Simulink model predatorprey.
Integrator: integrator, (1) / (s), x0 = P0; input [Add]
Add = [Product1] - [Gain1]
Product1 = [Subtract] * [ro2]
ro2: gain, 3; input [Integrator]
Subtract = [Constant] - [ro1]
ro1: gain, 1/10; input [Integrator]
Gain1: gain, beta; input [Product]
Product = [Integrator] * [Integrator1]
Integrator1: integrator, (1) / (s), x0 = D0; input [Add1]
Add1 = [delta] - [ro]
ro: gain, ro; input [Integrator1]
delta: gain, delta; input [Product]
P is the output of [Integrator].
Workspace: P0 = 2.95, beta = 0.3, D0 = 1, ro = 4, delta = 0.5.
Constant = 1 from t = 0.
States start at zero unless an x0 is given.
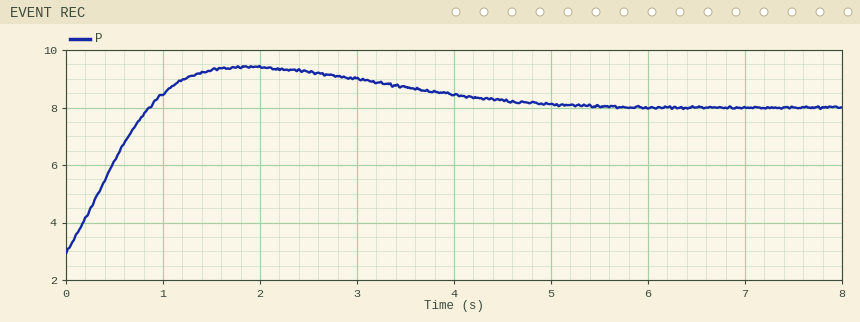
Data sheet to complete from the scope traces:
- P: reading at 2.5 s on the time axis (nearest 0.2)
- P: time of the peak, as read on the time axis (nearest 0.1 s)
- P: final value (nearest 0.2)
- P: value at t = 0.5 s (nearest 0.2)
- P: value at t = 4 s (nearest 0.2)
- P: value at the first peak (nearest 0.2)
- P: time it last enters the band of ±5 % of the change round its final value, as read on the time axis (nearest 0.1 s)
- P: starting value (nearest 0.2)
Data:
9.2
1.9 s
8.0
6.2
8.4
9.4
4.5 s
3.0
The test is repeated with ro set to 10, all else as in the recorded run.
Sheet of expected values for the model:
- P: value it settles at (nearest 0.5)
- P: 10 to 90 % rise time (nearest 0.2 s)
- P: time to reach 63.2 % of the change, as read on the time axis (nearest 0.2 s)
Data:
10.0
1.0 s
0.6 s
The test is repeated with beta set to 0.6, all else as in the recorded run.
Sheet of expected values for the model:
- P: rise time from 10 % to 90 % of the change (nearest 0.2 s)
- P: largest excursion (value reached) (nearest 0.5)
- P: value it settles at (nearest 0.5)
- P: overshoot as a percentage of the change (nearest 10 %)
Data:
0.8 s
9.0
8.0
20 %
